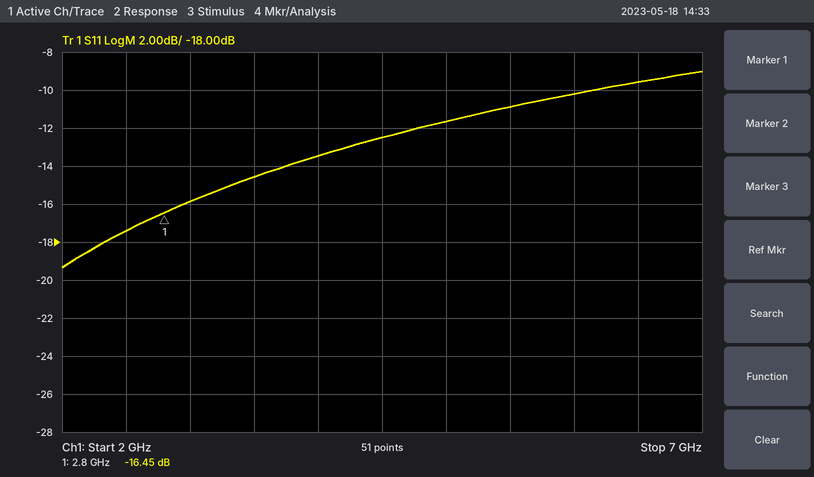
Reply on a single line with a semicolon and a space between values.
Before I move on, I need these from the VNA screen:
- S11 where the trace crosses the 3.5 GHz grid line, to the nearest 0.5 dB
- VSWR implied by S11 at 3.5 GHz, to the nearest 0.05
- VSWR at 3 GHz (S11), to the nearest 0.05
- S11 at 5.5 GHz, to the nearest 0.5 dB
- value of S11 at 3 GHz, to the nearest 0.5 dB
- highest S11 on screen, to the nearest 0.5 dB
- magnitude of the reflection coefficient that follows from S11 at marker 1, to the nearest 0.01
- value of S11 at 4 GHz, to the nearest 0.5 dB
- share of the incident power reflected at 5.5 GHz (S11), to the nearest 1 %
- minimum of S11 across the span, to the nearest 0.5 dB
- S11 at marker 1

-14.5 dB; 1.45; 1.40; -11.0 dB; -16.0 dB; -9.0 dB; 0.15; -13.5 dB; 8 %; -19.5 dB; -16.45 dB
